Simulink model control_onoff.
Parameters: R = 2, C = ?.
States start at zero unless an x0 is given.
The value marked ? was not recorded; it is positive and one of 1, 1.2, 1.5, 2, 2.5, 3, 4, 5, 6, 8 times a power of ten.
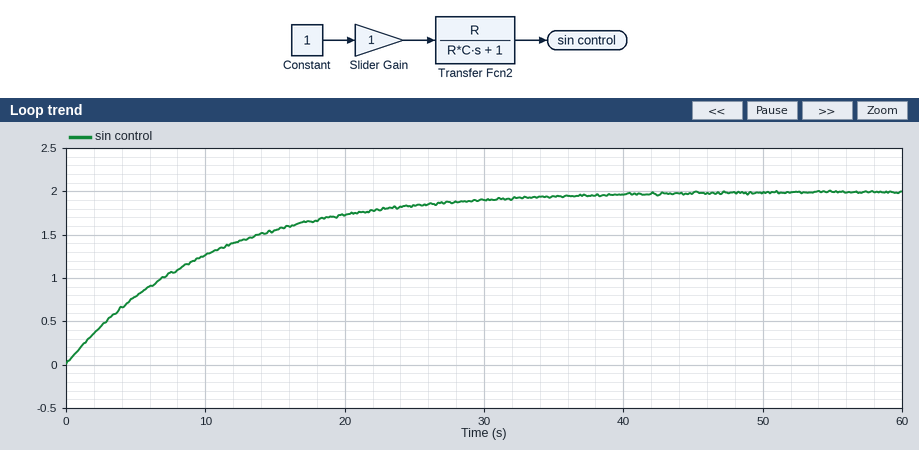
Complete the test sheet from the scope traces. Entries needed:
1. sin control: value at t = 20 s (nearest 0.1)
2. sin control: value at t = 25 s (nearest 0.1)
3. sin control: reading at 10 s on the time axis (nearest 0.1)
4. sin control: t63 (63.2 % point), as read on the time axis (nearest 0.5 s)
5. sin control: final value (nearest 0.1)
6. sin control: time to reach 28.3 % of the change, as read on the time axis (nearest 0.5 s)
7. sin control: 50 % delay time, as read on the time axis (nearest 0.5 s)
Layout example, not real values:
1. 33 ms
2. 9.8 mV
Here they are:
1. 1.7
2. 1.8
3. 1.3
4. 10.0 s
5. 2.0
6. 3.5 s
7. 7.0 s
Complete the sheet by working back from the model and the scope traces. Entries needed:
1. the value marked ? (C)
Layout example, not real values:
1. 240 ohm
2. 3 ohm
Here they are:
1. 5
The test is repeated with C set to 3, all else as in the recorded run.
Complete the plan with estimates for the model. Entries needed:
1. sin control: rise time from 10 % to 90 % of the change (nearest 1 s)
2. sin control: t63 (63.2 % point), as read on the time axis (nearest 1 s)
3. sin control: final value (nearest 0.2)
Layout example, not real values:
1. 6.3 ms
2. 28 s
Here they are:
1. 13 s
2. 6 s
3. 2.0
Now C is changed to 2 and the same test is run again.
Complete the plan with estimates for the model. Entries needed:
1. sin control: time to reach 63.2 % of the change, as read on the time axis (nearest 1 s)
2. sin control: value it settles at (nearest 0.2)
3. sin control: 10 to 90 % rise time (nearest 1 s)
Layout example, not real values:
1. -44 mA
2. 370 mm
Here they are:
1. 4 s
2. 2.0
3. 9 s
